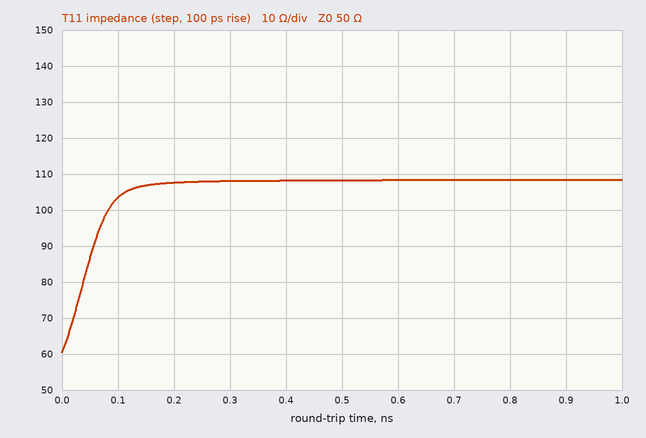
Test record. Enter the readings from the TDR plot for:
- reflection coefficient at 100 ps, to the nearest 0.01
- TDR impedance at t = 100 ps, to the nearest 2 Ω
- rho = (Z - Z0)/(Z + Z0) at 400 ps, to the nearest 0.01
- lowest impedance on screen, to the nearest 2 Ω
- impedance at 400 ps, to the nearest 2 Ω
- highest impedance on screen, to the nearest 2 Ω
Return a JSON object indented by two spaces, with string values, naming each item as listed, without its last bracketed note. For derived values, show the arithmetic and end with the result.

{
  "reflection coefficient at 100 ps, to the nearest 0.01": "(104 − 50)/(104 + 50) ≈ +0.35",
  "TDR impedance at t = 100 ps, to the nearest 2 Ω": "104 Ω",
  "rho = (Z - Z0)/(Z + Z0) at 400 ps, to the nearest 0.01": "(108 − 50)/(108 + 50) ≈ +0.37",
  "lowest impedance on screen, to the nearest 2 Ω": "60 Ω",
  "impedance at 400 ps, to the nearest 2 Ω": "108 Ω",
  "highest impedance on screen, to the nearest 2 Ω": "108 Ω"
}
